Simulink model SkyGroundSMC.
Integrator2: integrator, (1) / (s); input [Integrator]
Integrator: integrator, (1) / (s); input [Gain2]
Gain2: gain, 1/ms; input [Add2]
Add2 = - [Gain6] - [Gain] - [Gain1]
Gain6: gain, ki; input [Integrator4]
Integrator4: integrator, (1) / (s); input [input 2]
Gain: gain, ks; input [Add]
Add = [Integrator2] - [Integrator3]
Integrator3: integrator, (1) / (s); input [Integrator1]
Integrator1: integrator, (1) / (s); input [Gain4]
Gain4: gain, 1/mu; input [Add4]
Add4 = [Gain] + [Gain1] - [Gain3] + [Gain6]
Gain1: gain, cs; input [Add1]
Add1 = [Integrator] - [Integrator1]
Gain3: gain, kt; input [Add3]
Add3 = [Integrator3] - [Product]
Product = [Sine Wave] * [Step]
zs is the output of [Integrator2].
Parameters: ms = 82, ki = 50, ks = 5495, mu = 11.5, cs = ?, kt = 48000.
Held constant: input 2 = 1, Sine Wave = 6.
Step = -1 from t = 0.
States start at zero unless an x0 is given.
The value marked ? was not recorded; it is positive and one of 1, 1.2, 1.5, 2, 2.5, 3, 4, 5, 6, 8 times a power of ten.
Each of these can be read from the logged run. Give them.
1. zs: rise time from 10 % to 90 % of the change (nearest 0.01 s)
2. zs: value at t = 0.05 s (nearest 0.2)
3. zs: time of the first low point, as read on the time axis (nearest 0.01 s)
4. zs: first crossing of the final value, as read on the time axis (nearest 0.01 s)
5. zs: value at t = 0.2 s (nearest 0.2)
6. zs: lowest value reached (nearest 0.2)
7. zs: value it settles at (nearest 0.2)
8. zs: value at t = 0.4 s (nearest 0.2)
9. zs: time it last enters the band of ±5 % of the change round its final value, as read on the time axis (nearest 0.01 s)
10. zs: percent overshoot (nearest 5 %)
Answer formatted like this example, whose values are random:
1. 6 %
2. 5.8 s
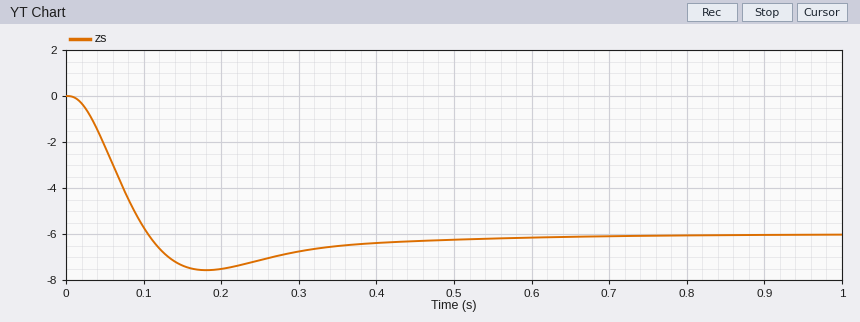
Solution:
1. 0.07 s
2. -2.2
3. 0.18 s
4. 0.11 s
5. -7.6
6. -7.6
7. -6.0
8. -6.4
9. 0.43 s
10. 25 %
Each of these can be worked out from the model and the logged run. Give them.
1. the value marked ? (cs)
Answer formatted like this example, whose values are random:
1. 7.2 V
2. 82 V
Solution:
1. 1500
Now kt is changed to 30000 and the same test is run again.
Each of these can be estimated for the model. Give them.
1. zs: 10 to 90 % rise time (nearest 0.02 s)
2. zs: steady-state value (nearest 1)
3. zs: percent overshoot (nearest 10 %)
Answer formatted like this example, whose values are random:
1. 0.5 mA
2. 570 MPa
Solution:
1. 0.08 s
2. -6
3. 40 %
